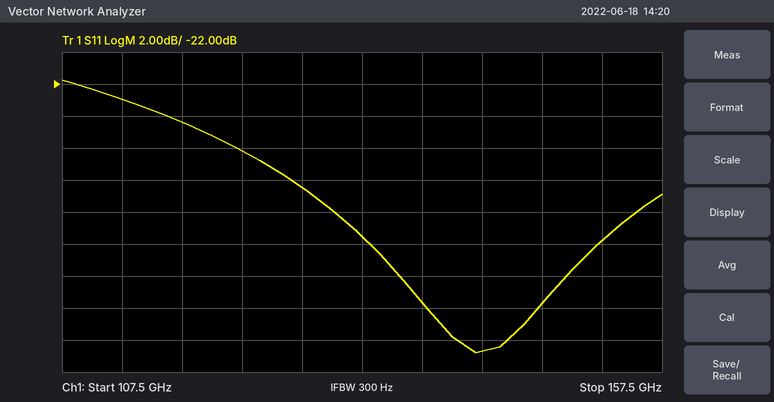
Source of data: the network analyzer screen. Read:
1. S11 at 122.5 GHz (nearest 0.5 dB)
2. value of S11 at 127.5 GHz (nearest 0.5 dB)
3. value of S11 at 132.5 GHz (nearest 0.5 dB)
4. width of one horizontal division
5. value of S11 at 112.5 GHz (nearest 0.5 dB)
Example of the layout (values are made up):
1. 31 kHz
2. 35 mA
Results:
1. -26.0 dB
2. -28.5 dB
3. -31.5 dB
4. 5 GHz
5. -23.0 dB
